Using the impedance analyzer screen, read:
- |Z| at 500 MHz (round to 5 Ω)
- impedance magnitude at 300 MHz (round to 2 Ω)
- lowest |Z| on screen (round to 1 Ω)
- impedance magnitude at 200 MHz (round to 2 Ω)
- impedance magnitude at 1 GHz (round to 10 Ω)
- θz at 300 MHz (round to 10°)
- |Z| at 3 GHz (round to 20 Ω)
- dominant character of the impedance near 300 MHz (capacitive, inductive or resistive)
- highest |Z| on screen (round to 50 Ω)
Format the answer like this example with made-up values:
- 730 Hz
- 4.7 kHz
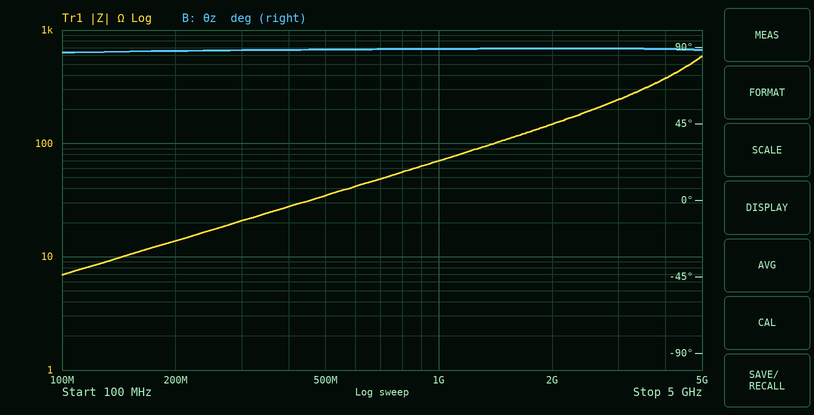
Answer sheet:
- 35 Ω
- 20 Ω
- 7 Ω
- 14 Ω
- 70 Ω
- 90°
- 240 Ω
- inductive
- 600 Ω
